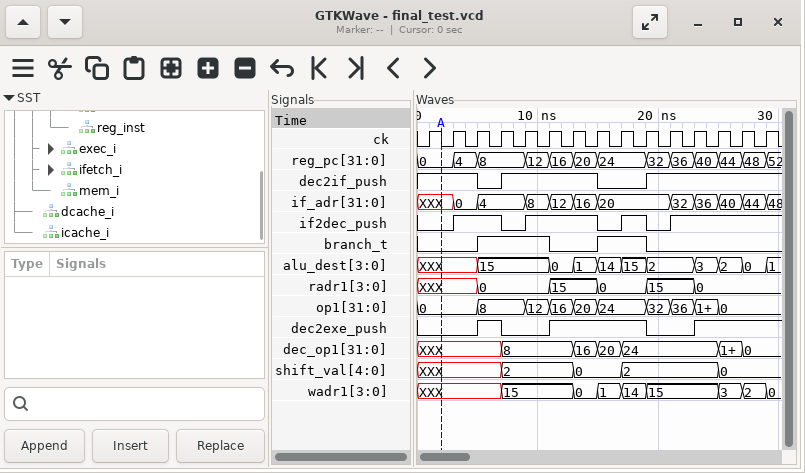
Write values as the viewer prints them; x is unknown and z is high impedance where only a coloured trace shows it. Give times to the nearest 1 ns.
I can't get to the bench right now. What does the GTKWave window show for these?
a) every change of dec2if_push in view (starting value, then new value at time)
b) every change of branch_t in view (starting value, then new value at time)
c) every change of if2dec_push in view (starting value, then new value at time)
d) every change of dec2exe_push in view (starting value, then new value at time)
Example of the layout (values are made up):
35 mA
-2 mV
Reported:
1, 0 at 5 ns, 1 at 7 ns, 0 at 15 ns, 1 at 19 ns
0, 1 at 5 ns, 0 at 11 ns, 1 at 15 ns, 0 at 19 ns
0, 1 at 3 ns, 0 at 7 ns, 1 at 9 ns, 0 at 15 ns, 1 at 17 ns, 0 at 19 ns, 1 at 21 ns
0, 1 at 5 ns, 0 at 7 ns, 1 at 11 ns, 0 at 19 ns, 1 at 23 ns
